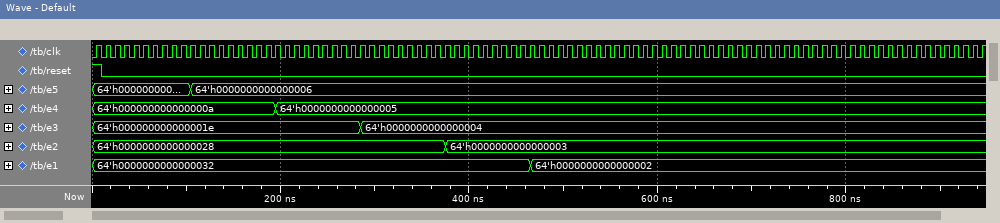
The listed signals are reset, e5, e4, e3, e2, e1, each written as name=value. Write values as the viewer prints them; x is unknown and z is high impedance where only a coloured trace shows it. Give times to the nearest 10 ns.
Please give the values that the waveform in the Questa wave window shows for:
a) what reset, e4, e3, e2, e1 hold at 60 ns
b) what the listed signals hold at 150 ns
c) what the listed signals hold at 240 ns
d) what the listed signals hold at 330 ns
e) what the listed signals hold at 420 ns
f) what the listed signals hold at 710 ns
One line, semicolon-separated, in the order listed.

reset=0, e4=64'h000000000000000a, e3=64'h000000000000001e, e2=64'h0000000000000028, e1=64'h0000000000000032; reset=0, e5=64'h0000000000000006, e4=64'h000000000000000a, e3=64'h000000000000001e, e2=64'h0000000000000028, e1=64'h0000000000000032; reset=0, e5=64'h0000000000000006, e4=64'h0000000000000005, e3=64'h000000000000001e, e2=64'h0000000000000028, e1=64'h0000000000000032; reset=0, e5=64'h0000000000000006, e4=64'h0000000000000005, e3=64'h0000000000000004, e2=64'h0000000000000028, e1=64'h0000000000000032; reset=0, e5=64'h0000000000000006, e4=64'h0000000000000005, e3=64'h0000000000000004, e2=64'h0000000000000003, e1=64'h0000000000000032; reset=0, e5=64'h0000000000000006, e4=64'h0000000000000005, e3=64'h0000000000000004, e2=64'h0000000000000003, e1=64'h0000000000000002
